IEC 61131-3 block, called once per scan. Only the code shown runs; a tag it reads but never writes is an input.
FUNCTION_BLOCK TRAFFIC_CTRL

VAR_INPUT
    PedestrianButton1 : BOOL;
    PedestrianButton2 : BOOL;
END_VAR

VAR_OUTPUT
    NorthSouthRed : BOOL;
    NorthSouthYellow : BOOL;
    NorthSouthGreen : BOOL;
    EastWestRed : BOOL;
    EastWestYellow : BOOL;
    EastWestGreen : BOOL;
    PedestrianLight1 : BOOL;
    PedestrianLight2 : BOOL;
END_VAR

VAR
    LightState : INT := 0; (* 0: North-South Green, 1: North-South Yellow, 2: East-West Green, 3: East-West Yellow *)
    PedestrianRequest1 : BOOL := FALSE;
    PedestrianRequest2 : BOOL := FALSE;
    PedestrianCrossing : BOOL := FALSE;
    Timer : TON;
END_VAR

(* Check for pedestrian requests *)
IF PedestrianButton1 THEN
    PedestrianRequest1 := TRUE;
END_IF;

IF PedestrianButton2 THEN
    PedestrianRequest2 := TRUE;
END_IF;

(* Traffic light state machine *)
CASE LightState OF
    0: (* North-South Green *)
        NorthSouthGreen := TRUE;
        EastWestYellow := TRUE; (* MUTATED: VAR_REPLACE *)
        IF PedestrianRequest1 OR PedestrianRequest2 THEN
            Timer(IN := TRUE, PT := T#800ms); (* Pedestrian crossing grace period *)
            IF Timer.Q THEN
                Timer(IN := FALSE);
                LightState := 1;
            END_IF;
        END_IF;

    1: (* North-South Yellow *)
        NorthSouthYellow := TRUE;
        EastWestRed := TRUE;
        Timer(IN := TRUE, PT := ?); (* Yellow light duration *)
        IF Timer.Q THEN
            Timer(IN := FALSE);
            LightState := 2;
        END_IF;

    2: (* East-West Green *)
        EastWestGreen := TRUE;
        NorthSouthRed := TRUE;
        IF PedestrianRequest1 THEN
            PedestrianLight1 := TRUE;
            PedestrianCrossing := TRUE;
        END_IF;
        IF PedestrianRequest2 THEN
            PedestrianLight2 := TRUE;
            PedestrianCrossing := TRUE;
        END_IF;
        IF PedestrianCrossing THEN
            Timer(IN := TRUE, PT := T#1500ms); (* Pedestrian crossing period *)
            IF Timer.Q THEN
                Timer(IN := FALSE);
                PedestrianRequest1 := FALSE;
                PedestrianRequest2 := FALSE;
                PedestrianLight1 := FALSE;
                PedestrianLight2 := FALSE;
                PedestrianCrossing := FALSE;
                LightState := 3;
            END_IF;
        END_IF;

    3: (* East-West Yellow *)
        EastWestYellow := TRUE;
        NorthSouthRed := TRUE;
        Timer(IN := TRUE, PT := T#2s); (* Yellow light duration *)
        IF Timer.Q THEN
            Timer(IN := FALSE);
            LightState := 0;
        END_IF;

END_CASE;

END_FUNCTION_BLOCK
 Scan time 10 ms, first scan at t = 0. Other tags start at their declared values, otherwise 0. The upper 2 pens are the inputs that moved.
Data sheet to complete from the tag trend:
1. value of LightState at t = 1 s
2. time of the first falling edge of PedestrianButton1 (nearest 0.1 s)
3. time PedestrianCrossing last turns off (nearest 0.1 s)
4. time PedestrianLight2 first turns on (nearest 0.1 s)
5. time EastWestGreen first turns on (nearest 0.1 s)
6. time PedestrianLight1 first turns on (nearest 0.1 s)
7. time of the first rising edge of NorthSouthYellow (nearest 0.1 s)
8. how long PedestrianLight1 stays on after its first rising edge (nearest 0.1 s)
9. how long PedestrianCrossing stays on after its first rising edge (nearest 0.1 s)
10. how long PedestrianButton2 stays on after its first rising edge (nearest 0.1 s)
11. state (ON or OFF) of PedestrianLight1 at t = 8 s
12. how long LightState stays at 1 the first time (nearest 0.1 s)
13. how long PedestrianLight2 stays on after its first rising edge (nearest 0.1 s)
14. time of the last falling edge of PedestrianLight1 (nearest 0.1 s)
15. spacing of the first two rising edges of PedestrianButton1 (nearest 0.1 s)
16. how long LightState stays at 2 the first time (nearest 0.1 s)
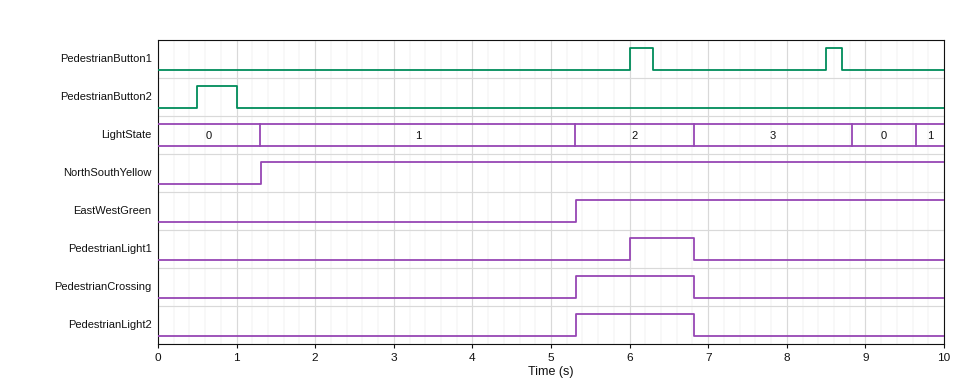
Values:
0
6.3 s
6.8 s
5.3 s
5.3 s
6.0 s
1.3 s
0.8 s
1.5 s
0.5 s
OFF
4.0 s
1.5 s
6.8 s
2.5 s
1.5 s
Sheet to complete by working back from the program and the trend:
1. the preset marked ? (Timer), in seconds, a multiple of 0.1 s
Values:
4.0 s
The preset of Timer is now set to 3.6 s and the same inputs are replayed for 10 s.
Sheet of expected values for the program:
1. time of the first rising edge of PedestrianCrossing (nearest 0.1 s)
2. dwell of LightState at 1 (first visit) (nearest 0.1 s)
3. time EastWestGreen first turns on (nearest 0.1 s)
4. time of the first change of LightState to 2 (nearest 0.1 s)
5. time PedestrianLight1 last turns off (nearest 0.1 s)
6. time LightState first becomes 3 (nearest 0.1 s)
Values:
4.9 s
3.6 s
4.9 s
4.9 s
6.4 s
6.4 s
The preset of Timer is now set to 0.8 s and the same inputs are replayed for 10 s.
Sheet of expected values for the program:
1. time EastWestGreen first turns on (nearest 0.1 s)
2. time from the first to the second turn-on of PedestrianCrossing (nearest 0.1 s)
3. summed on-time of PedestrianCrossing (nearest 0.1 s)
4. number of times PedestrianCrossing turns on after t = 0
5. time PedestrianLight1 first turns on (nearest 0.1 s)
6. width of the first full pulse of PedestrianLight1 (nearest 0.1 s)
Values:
2.1 s
5.5 s
3.0 s
2
7.6 s
1.5 s
